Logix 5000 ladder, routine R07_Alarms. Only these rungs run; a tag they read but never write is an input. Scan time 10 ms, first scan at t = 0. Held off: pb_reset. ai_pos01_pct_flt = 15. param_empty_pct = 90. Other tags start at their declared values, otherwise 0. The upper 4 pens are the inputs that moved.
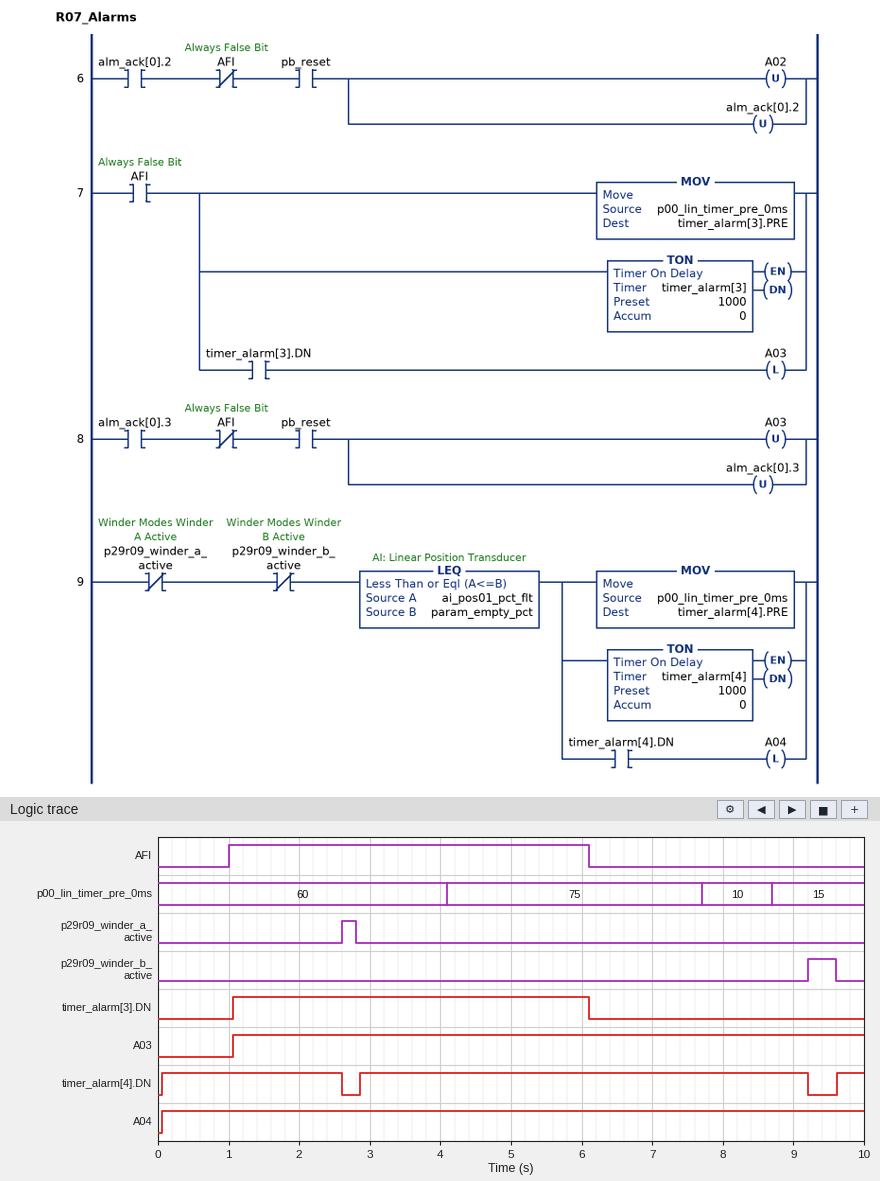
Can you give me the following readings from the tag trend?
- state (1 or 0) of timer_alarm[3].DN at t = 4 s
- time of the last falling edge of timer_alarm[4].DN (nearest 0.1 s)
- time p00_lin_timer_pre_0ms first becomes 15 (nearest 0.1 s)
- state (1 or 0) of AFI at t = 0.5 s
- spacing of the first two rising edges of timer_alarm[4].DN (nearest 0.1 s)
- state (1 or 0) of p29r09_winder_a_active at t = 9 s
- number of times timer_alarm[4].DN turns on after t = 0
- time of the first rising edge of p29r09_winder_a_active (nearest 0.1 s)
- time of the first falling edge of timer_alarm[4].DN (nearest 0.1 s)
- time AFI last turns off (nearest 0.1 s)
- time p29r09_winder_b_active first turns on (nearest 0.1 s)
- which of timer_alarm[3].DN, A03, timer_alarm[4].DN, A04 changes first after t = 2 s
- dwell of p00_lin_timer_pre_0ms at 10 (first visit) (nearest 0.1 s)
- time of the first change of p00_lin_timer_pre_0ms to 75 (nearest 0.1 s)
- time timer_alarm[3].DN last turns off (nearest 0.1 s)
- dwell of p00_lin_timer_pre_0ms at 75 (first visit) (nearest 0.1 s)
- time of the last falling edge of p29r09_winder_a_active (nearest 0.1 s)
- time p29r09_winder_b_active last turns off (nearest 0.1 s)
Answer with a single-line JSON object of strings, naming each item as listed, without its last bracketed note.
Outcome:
{"state (1 or 0) of timer_alarm[3].DN at t = 4 s": "1", "time of the last falling edge of timer_alarm[4].DN": "9.2 s", "time p00_lin_timer_pre_0ms first becomes 15": "8.7 s", "state (1 or 0) of AFI at t = 0.5 s": "0", "spacing of the first two rising edges of timer_alarm[4].DN": "2.8 s", "state (1 or 0) of p29r09_winder_a_active at t = 9 s": "0", "number of times timer_alarm[4].DN turns on after t = 0": "3", "time of the first rising edge of p29r09_winder_a_active": "2.6 s", "time of the first falling edge of timer_alarm[4].DN": "2.6 s", "time AFI last turns off": "6.1 s", "time p29r09_winder_b_active first turns on": "9.2 s", "which of timer_alarm[3].DN, A03, timer_alarm[4].DN, A04 changes first after t = 2 s": "timer_alarm[4].DN", "dwell of p00_lin_timer_pre_0ms at 10 (first visit)": "1.0 s", "time of the first change of p00_lin_timer_pre_0ms to 75": "4.1 s", "time timer_alarm[3].DN last turns off": "6.1 s", "dwell of p00_lin_timer_pre_0ms at 75 (first visit)": "3.6 s", "time of the last falling edge of p29r09_winder_a_active": "2.8 s", "time p29r09_winder_b_active last turns off": "9.6 s"}
